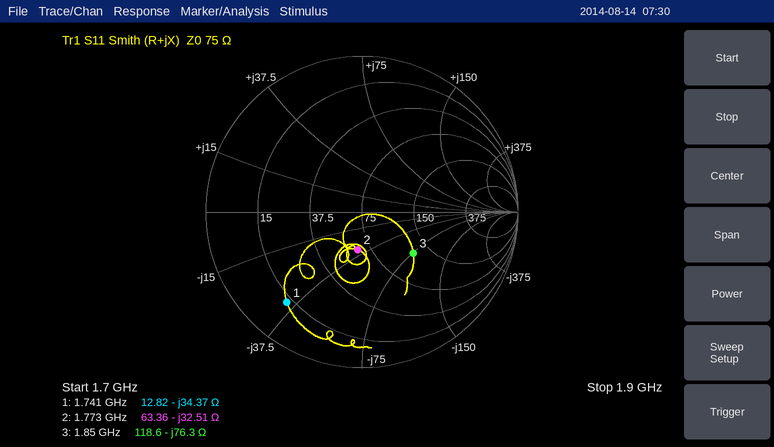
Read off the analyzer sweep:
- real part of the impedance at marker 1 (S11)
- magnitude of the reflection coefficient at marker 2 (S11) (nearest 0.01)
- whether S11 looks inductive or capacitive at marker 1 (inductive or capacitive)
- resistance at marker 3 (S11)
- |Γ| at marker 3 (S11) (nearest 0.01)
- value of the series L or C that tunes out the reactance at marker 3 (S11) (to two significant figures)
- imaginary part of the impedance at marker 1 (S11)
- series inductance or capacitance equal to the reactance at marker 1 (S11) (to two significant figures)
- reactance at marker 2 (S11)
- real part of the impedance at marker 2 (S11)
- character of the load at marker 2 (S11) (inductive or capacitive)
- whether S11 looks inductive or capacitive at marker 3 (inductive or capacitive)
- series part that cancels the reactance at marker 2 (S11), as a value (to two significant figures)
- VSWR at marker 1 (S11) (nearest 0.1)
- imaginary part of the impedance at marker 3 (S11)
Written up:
12.82 Ω
0.24
capacitive
118.6 Ω
0.42
6.6 nH
-34.37 Ω
2.7 pF
-32.51 Ω
63.36 Ω
capacitive
capacitive
2.9 nH
7.1
-76.3 Ω
